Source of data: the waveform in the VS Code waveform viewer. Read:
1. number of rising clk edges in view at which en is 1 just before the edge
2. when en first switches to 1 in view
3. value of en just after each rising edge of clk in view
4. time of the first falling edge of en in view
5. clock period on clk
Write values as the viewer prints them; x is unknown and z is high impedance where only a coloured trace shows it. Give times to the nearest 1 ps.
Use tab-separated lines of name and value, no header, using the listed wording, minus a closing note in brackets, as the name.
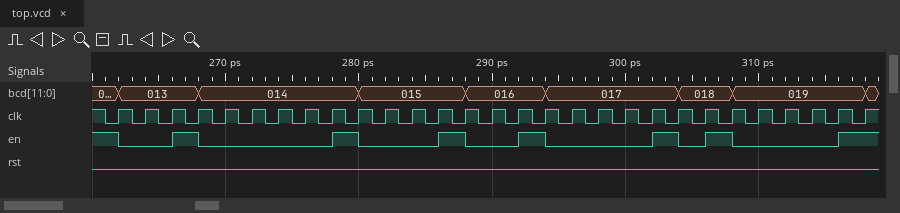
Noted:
number of rising clk edges in view at which en is 1 just before the edge	8
when en first switches to 1 in view	266 ps
value of en just after each rising edge of clk in view	0 0 1 0 0 0 0 0 1 0 0 0 1 0 0 1 0 0 0 0 1 0 1 0 0 0 0 1 1
time of the first falling edge of en in view	262 ps
clock period on clk	2 ps
